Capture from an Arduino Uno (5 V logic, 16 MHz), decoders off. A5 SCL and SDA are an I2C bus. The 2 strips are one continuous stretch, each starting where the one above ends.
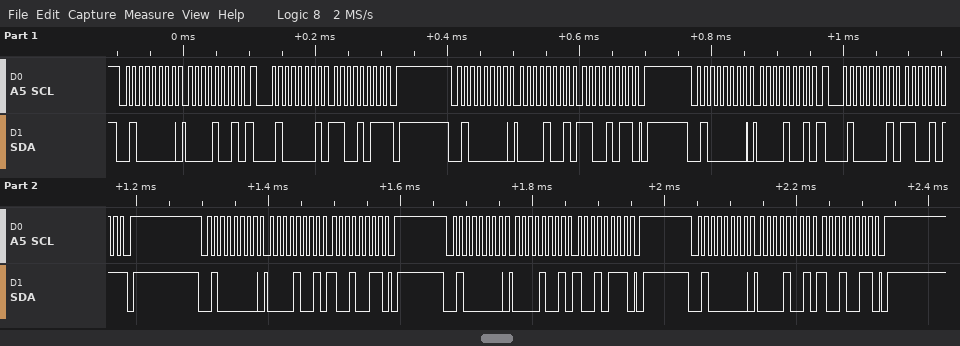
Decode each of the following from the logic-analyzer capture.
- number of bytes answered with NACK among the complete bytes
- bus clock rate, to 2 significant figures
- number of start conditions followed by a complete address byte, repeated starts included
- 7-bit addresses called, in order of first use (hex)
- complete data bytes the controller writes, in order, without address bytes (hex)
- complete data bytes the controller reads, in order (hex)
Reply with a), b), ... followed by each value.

a) 2
b) 100 kHz
c) 8
d) 0x20
e) 09 09 CB 09 09 93 09 97 09 93
f) CB CB
